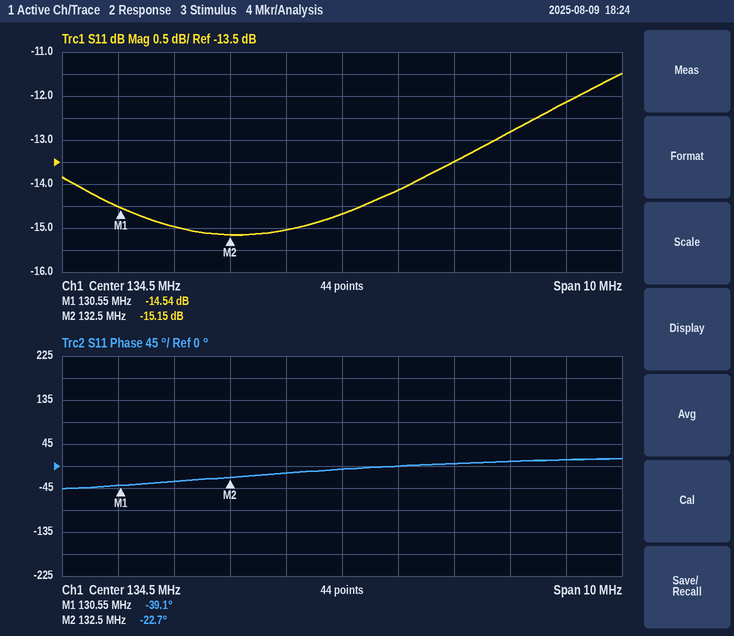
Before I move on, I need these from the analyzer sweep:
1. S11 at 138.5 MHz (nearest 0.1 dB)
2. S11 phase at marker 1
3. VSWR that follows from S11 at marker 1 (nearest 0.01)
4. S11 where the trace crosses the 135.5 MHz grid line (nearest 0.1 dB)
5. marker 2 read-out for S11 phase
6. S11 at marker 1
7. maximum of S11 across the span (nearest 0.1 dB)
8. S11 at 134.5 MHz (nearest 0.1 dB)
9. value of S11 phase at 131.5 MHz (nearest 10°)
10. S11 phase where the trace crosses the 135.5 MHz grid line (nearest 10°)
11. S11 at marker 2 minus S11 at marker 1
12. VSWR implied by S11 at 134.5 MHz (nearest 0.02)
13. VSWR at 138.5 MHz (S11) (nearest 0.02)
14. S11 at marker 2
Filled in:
-12.1 dB
-39.1°
1.46
-14.1 dB
-22.7°
-14.54 dB
-11.5 dB
-14.7 dB
-30°
0°
-0.61 dB
1.46
1.66
-15.15 dB
